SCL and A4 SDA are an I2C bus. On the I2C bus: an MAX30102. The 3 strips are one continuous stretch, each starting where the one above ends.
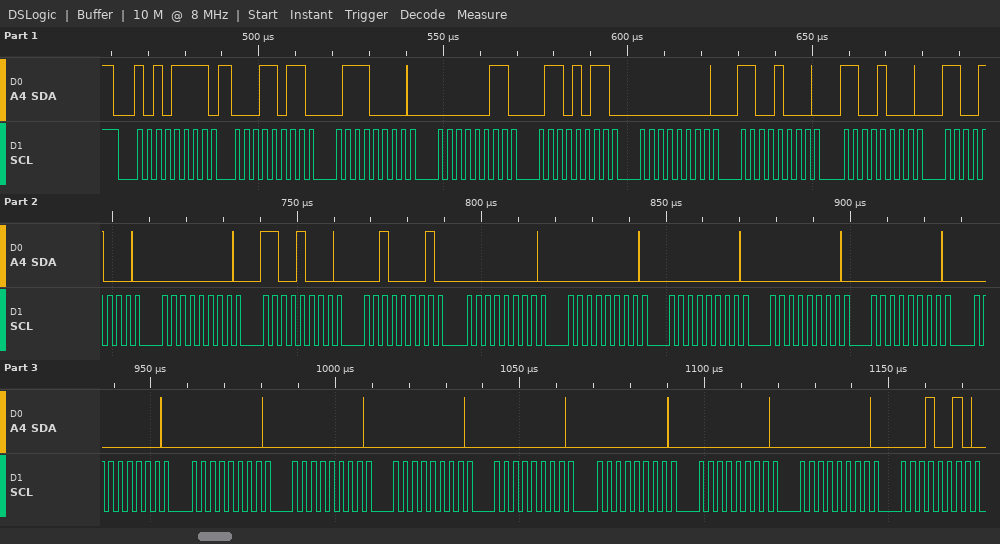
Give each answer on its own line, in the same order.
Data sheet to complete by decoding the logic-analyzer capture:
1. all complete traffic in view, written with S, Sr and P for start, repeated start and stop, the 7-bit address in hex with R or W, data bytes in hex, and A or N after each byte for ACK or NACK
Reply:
S 57R A 1B A 70 A 03 A 6B A 00 A C8 A C8 A C8 A 00 A C8 A 21 A 00 A 00 A 00 A 00 A 00 A 00 A 00 A 00 A 00 A 00 A 00 A 00 A 00 A 12 A
